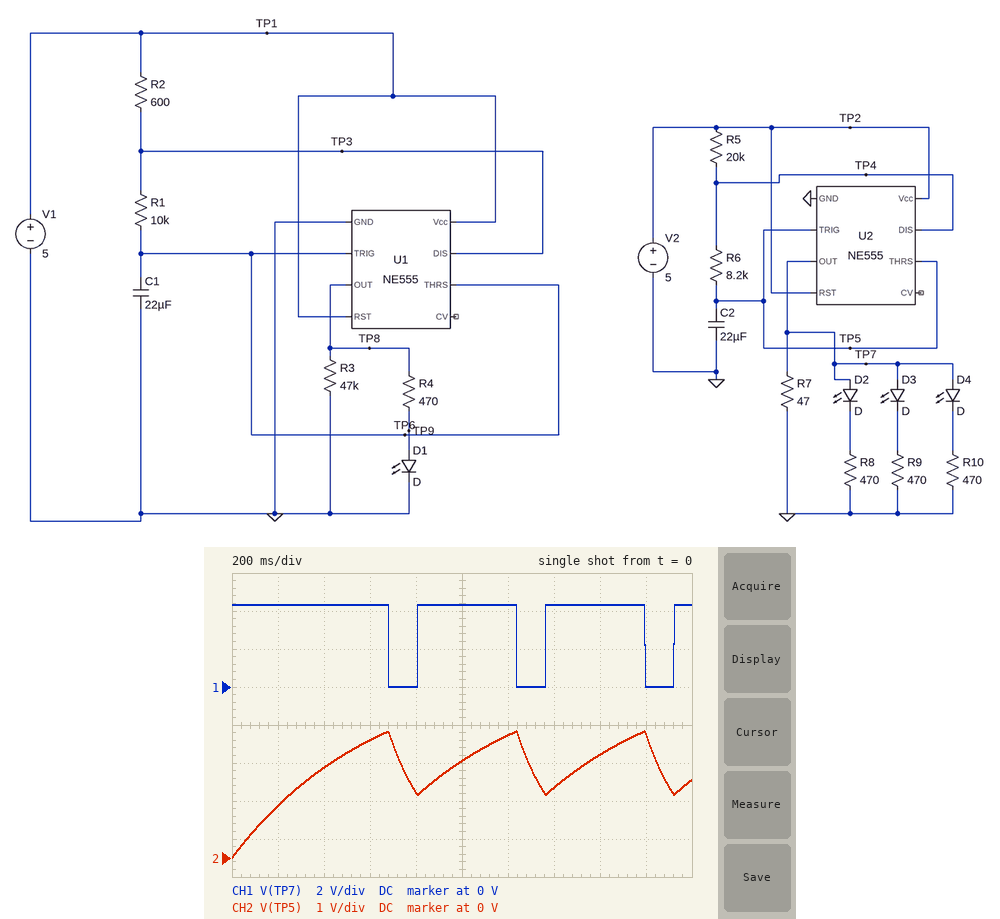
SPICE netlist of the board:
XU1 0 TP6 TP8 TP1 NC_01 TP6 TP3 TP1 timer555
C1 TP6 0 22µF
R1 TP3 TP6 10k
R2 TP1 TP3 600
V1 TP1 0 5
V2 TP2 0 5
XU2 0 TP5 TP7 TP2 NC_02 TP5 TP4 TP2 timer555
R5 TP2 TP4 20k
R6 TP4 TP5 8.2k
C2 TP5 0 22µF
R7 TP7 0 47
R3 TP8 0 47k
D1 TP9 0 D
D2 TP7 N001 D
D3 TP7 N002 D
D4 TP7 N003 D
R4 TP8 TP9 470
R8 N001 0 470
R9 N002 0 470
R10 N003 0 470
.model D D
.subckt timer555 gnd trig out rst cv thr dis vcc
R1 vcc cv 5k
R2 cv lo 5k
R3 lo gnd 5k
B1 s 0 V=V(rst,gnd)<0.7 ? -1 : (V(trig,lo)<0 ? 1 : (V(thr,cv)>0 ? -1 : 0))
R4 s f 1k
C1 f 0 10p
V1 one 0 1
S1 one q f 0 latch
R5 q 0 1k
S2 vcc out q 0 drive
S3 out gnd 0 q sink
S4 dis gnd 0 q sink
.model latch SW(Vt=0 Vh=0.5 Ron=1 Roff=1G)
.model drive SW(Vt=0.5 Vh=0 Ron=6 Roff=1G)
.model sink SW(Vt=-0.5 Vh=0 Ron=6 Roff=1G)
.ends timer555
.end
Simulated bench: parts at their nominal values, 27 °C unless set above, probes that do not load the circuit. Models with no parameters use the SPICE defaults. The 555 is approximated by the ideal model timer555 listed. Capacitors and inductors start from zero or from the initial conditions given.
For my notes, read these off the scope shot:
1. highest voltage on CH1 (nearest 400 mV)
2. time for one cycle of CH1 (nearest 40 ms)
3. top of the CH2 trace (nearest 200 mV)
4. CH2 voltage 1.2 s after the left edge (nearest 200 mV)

4.4 V
560 ms
3.4 V
3.2 V
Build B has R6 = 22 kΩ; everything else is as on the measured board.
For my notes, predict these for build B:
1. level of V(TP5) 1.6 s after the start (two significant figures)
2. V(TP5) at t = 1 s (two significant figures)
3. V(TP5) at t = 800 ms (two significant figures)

2.5 V
3.3 V
2.9 V
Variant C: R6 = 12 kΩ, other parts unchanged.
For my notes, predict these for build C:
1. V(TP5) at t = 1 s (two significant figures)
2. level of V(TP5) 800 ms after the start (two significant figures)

1.9 V
3.0 V
